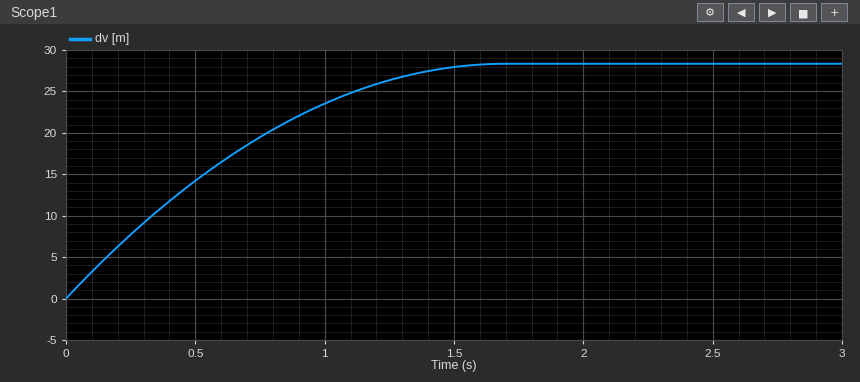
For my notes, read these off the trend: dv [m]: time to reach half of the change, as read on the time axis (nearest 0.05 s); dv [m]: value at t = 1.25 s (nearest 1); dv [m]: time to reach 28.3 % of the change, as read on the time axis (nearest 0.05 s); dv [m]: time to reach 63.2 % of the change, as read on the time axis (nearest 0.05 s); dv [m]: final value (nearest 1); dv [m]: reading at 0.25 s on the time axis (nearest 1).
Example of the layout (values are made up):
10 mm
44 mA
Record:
0.50 s
26
0.25 s
0.65 s
28
8
